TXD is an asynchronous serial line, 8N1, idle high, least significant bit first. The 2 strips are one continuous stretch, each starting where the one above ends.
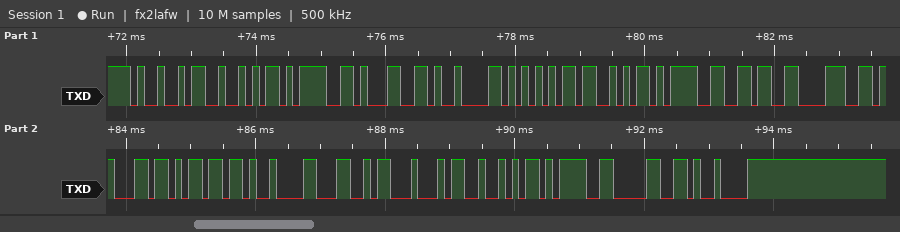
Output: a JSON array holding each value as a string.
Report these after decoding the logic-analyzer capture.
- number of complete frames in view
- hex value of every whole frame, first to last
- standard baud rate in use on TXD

["19", "0x49 0x52 0x3D 0x31 0x09 0x55 0x53 0x3D 0x36 0x38 0x63 0x6D 0x09 0x4C 0x44 0x52 0x3D 0x30 0x09", "9600 baud"]
